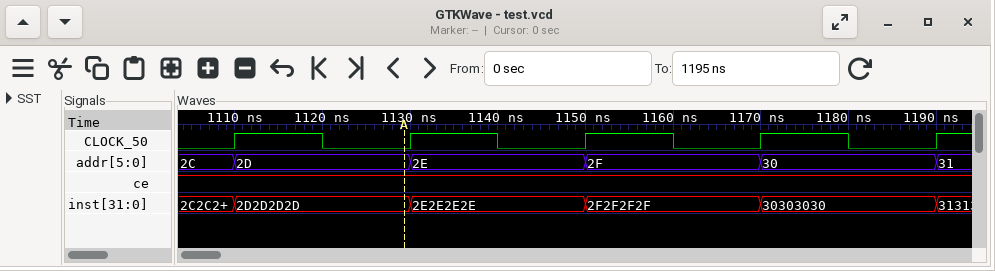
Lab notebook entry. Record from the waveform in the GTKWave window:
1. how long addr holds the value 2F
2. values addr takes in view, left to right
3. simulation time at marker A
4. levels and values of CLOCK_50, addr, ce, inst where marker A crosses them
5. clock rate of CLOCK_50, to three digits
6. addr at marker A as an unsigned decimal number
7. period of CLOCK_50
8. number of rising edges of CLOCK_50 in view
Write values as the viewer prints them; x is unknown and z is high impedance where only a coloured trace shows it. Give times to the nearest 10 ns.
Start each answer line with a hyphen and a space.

- 20 ns
- 2C, 2D, 2E, 2F, 30, 31
- 1130 ns
- CLOCK_50=0, addr=2D, ce=1, inst=2D2D2D2D
- 50.0 MHz
- 45
- 20 ns
- 5
